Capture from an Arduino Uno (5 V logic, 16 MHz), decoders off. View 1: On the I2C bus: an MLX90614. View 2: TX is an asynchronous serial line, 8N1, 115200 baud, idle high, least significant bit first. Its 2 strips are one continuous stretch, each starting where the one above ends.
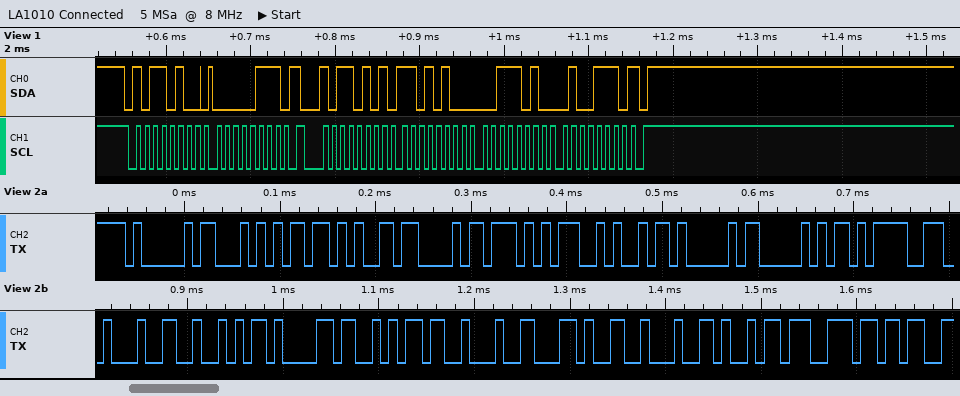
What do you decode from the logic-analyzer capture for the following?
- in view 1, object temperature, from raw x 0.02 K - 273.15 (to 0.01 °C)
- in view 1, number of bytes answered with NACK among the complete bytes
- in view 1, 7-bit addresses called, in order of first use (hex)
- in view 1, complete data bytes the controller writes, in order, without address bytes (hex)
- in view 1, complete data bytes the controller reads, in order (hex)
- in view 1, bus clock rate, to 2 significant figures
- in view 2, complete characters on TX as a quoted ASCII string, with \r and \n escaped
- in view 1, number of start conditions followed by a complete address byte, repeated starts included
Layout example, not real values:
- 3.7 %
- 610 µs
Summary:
- 28.05 °C
- 1
- 0x5A
- 07
- D4 3A 4E
- 100 kHz
- "AT+CWJAP=\"Raj\",\"in"
- 2
